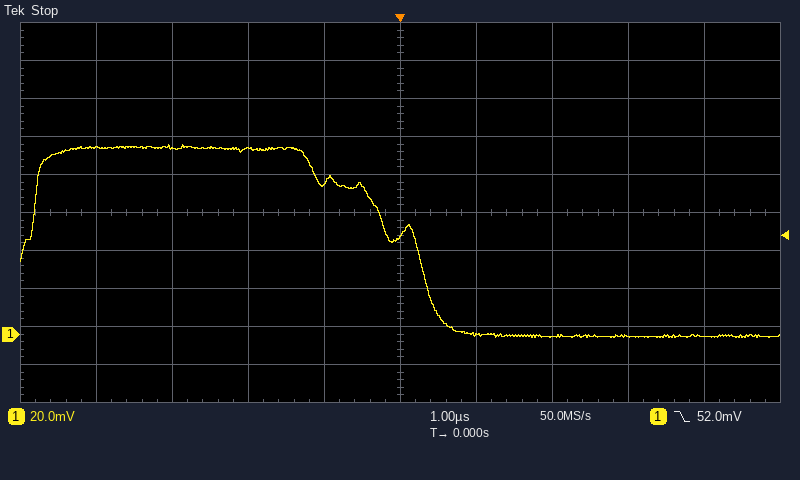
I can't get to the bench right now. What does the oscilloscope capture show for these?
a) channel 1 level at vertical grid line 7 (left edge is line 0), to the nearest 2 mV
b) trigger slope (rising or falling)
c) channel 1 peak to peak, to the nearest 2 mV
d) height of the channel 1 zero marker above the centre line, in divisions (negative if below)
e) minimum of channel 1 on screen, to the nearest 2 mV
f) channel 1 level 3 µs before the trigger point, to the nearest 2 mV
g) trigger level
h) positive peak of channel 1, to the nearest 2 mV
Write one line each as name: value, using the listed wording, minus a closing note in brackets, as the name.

channel 1 level at vertical grid line 7 (left edge is line 0), to the nearest 2 mV: -2 mV
trigger slope: falling
channel 1 peak to peak, to the nearest 2 mV: 102 mV
height of the channel 1 zero marker above the centre line, in divisions: -3.2 div
minimum of channel 1 on screen, to the nearest 2 mV: -2 mV
channel 1 level 3 µs before the trigger point, to the nearest 2 mV: 98 mV
trigger level: 52.0 mV
positive peak of channel 1, to the nearest 2 mV: 100 mV
